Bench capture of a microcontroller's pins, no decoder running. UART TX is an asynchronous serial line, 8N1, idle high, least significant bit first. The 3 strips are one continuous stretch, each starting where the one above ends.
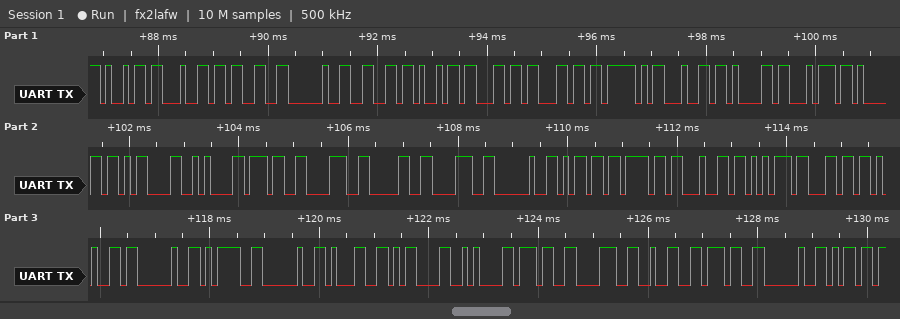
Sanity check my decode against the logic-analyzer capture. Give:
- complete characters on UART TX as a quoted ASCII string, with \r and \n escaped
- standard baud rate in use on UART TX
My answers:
"id3 fill_data\r\n7808 module = 1\r\n7827 m"
9600 baud
